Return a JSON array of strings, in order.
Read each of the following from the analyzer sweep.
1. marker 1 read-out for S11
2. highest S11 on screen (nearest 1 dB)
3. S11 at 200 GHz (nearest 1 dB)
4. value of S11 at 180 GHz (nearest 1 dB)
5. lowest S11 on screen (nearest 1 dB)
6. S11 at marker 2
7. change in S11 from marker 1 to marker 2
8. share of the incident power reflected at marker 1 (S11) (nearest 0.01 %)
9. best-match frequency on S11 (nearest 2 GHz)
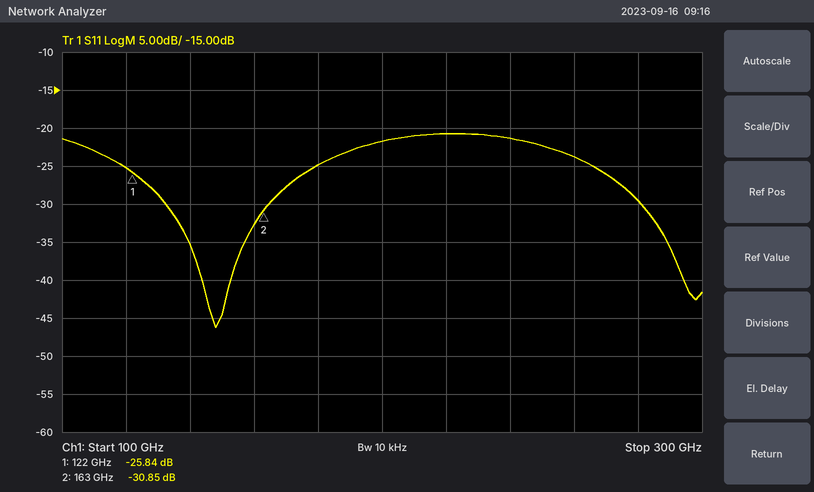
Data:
["-25.84 dB", "-21 dB", "-22 dB", "-25 dB", "-46 dB", "-30.85 dB", "-5.01 dB", "0.26 %", "148 GHz"]
